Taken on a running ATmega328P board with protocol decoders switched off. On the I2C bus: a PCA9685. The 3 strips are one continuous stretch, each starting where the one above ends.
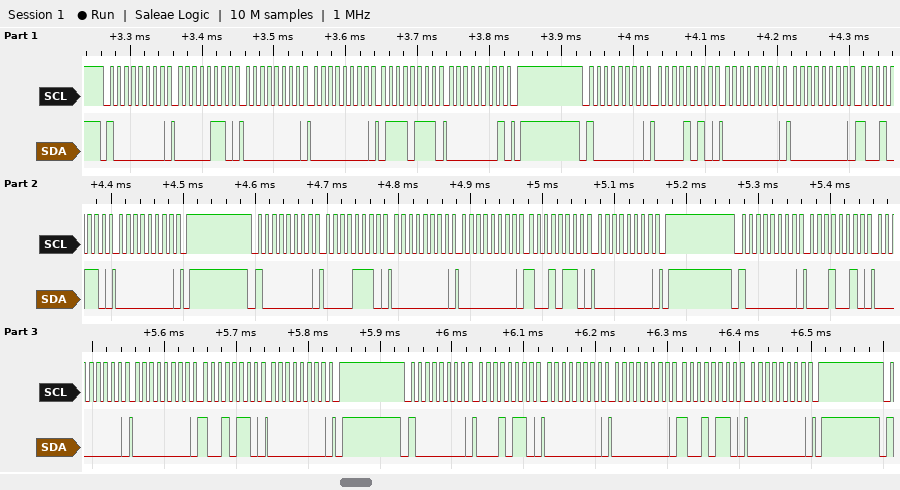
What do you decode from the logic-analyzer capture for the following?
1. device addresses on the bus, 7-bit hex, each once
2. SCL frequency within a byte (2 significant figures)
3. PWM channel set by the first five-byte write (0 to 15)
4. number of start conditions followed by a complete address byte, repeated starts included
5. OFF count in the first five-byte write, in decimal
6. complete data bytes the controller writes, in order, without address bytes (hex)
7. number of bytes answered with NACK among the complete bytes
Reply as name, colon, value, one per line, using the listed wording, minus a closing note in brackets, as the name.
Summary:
device addresses on the bus, 7-bit hex, each once: 0x40
SCL frequency within a byte: 100 kHz
PWM channel set by the first five-byte write: 0
number of start conditions followed by a complete address byte, repeated starts included: 5
OFF count in the first five-byte write, in decimal: 375
complete data bytes the controller writes, in order, without address bytes: 06 00 00 77 01 0A 00 00 96 00 0E 00 00 96 00 12 00 00 96 00 16 00 00 96 00
number of bytes answered with NACK among the complete bytes: 0
